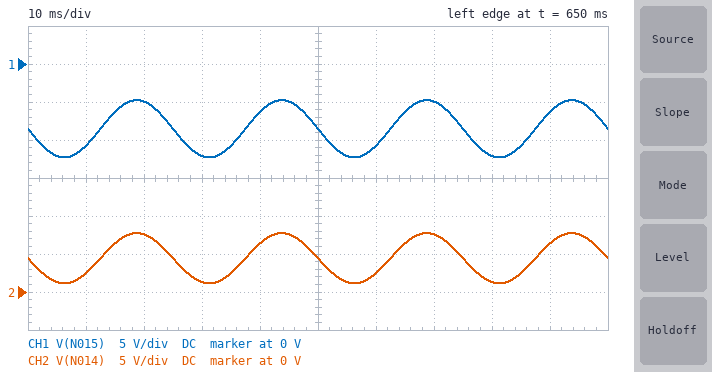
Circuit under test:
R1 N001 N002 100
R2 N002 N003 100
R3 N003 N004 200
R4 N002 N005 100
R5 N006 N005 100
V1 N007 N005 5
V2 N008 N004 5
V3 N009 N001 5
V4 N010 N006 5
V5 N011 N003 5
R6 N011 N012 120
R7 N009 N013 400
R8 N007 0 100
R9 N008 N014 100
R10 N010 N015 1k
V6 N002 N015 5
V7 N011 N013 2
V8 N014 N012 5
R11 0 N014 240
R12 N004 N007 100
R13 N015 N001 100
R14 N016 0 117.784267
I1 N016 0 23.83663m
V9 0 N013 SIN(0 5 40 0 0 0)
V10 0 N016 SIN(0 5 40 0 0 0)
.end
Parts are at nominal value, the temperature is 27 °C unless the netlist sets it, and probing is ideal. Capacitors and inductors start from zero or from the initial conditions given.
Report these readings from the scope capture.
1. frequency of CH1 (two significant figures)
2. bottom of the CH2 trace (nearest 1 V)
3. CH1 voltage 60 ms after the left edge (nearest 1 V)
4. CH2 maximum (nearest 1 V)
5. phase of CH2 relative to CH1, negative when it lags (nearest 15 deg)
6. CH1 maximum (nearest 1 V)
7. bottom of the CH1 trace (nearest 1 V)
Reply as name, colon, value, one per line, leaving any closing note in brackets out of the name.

frequency of CH1: 40 Hz
bottom of the CH2 trace: 1 V
CH1 voltage 60 ms after the left edge: -11 V
CH2 maximum: 8 V
phase of CH2 relative to CH1, negative when it lags: 0 deg
CH1 maximum: -5 V
bottom of the CH1 trace: -12 V
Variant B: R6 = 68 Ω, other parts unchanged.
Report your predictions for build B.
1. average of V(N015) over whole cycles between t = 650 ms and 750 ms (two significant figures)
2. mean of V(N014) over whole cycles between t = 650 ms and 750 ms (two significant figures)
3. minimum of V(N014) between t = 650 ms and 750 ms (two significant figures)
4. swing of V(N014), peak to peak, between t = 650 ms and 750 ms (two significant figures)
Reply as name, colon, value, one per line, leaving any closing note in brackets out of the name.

average of V(N015) over whole cycles between t = 650 ms and 750 ms: -8.5 V
mean of V(N014) over whole cycles between t = 650 ms and 750 ms: 5.1 V
minimum of V(N014) between t = 650 ms and 750 ms: 1.4 V
swing of V(N014), peak to peak, between t = 650 ms and 750 ms: 7.5 V
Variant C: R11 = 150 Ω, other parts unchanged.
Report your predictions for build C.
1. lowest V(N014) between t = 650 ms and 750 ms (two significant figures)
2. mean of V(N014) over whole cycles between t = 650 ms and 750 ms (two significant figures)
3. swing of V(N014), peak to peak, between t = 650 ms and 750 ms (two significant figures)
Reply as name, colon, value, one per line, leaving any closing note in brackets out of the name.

lowest V(N014) between t = 650 ms and 750 ms: 990 mV
mean of V(N014) over whole cycles between t = 650 ms and 750 ms: 3.9 V
swing of V(N014), peak to peak, between t = 650 ms and 750 ms: 5.8 V
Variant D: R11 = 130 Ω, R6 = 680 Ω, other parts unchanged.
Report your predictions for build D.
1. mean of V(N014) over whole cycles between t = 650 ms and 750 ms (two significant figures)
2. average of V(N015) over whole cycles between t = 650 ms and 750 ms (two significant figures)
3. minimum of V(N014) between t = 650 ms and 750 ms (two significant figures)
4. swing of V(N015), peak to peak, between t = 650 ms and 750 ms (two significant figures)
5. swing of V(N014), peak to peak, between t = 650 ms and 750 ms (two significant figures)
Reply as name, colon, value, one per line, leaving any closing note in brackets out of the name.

mean of V(N014) over whole cycles between t = 650 ms and 750 ms: 2.1 V
average of V(N015) over whole cycles between t = 650 ms and 750 ms: -8.7 V
minimum of V(N014) between t = 650 ms and 750 ms: 440 mV
swing of V(N015), peak to peak, between t = 650 ms and 750 ms: 7.3 V
swing of V(N014), peak to peak, between t = 650 ms and 750 ms: 3.4 V
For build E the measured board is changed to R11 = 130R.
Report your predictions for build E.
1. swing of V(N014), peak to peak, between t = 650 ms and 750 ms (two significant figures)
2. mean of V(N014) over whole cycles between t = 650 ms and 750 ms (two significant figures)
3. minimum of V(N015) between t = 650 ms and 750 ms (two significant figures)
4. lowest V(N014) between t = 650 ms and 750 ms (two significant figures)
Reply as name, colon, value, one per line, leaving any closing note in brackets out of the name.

swing of V(N014), peak to peak, between t = 650 ms and 750 ms: 5.5 V
mean of V(N014) over whole cycles between t = 650 ms and 750 ms: 3.7 V
minimum of V(N015) between t = 650 ms and 750 ms: -12 V
lowest V(N014) between t = 650 ms and 750 ms: 940 mV
